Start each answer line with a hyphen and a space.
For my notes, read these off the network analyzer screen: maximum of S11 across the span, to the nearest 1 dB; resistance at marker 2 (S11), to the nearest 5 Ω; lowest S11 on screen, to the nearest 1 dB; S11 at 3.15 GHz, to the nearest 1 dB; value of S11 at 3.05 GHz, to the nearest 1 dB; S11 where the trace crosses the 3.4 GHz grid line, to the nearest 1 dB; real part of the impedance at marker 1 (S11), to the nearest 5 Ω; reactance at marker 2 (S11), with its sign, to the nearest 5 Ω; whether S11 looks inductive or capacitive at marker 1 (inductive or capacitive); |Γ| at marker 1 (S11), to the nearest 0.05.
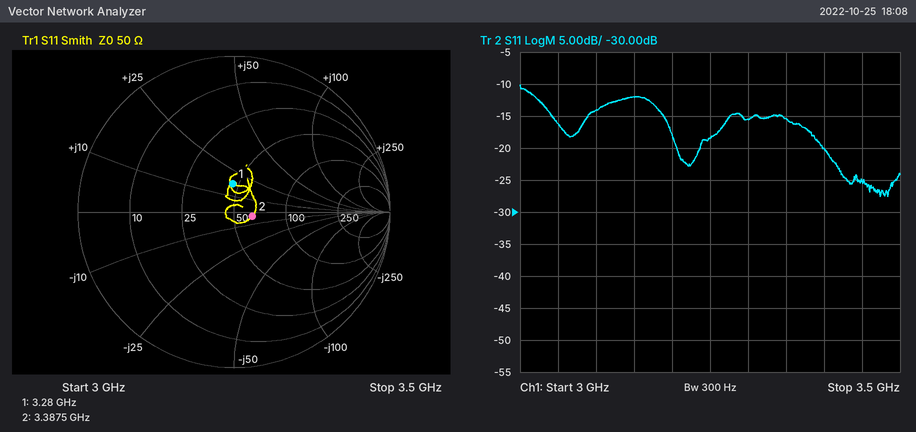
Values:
- -10 dB
- 65 Ω
- -28 dB
- -12 dB
- -16 dB
- -20 dB
- 45 Ω
- -5 Ω
- inductive
- 0.20
